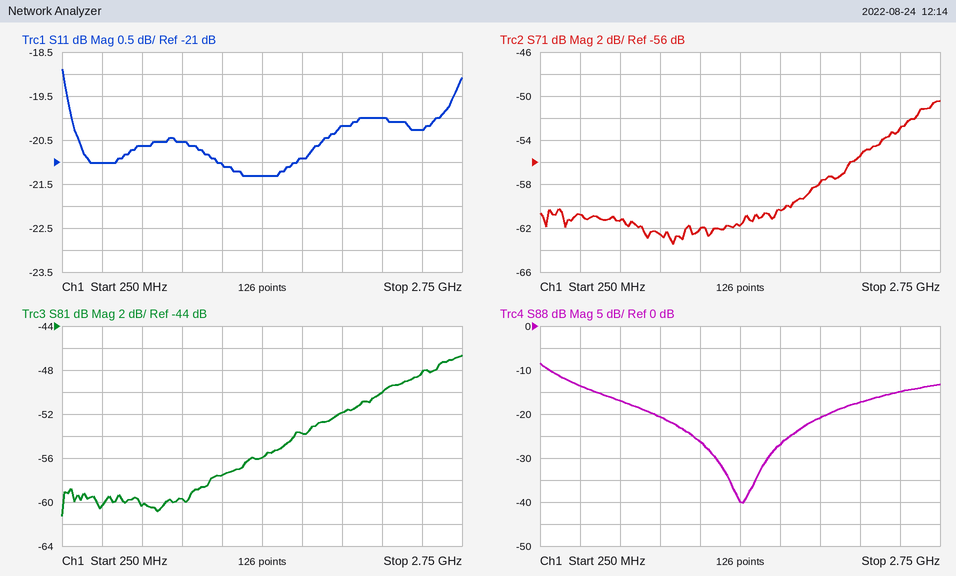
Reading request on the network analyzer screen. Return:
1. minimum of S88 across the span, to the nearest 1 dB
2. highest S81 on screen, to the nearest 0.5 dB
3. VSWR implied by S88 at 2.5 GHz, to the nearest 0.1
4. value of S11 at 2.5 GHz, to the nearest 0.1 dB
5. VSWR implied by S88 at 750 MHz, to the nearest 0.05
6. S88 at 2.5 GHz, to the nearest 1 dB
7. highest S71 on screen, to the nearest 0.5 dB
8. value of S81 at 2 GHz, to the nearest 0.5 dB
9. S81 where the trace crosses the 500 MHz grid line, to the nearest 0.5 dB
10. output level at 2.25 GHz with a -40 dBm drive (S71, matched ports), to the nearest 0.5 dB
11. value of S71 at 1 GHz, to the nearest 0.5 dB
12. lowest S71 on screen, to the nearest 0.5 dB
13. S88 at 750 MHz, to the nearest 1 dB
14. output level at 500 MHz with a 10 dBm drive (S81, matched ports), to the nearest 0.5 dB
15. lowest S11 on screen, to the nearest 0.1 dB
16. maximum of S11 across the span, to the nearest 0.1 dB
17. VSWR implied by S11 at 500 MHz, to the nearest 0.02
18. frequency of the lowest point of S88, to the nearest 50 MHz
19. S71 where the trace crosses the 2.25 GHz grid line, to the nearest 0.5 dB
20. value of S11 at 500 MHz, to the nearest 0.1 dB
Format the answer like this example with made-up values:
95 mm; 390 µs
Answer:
-40 dB; -46.5 dB; 1.4; -20.3 dB; 1.35; -15 dB; -50.5 dB; -52.0 dB; -60.5 dB; -95.5 dBm; -62.5 dB; -63.5 dB; -17 dB; -50.5 dBm; -21.3 dB; -18.9 dB; 1.20; 1.50 GHz; -55.5 dB; -21.0 dB
